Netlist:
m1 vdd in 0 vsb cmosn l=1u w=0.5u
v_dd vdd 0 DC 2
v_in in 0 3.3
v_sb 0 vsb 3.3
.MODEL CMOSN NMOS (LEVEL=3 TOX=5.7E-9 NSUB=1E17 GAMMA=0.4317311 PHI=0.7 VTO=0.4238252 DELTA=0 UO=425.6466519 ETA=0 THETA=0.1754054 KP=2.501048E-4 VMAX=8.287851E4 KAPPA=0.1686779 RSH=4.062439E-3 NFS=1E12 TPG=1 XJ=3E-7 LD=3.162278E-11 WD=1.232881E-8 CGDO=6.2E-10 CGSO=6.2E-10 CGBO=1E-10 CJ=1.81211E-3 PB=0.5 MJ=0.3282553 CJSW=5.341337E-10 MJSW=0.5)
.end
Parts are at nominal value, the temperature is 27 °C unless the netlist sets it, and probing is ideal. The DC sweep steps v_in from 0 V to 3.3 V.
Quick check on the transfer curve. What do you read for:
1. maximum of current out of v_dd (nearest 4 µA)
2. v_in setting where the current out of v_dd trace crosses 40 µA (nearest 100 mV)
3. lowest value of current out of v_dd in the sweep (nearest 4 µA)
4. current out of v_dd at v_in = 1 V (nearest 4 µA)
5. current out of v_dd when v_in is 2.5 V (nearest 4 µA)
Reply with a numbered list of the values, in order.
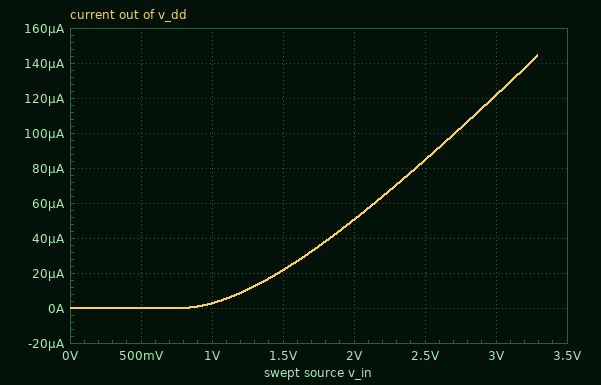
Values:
1. 144 µA
2. 1.8 V
3. 0 A
4. 4 µA
5. 84 µA
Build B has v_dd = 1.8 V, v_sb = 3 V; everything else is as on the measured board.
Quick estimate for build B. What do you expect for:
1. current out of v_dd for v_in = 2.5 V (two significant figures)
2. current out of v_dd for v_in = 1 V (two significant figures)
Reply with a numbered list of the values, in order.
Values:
1. 86 µA
2. 3.2 µA
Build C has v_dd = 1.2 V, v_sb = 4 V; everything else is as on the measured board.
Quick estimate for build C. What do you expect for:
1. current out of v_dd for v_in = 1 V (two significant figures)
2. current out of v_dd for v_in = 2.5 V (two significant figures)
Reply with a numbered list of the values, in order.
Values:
1. 1.7 µA
2. 79 µA
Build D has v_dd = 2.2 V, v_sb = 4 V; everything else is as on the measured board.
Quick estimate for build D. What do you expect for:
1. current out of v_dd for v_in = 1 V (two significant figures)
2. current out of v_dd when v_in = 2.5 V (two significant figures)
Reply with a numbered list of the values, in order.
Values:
1. 1.7 µA
2. 82 µA
